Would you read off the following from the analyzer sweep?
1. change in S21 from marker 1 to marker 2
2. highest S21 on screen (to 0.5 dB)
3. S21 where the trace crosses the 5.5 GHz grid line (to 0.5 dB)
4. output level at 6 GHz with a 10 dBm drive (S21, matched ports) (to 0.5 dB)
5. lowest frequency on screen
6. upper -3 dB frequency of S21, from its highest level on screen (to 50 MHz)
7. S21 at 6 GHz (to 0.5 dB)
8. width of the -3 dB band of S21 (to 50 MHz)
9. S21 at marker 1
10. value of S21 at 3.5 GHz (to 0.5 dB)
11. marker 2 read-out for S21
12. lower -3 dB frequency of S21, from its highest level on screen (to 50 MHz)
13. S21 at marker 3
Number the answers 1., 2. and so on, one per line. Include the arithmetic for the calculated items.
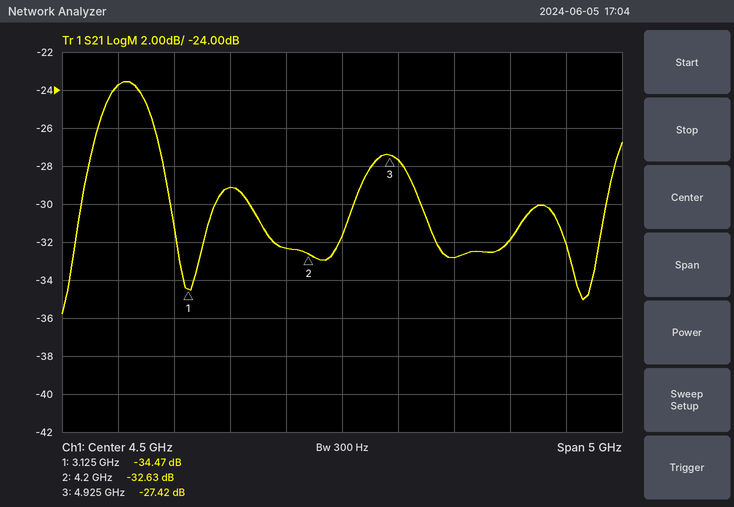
1. -32.63 − (-34.47) = 1.84 dB
2. -23.5 dB
3. -33.0 dB
4. 10 dBm + (-32.0 dB) = -22.0 dBm
5. 2 GHz
6. 2.85 GHz
7. -32.0 dB
8. 2.85 GHz − 2.30 GHz = 550 MHz
9. -34.47 dB
10. -29.0 dB
11. -32.63 dB
12. 2.30 GHz
13. -27.42 dB
